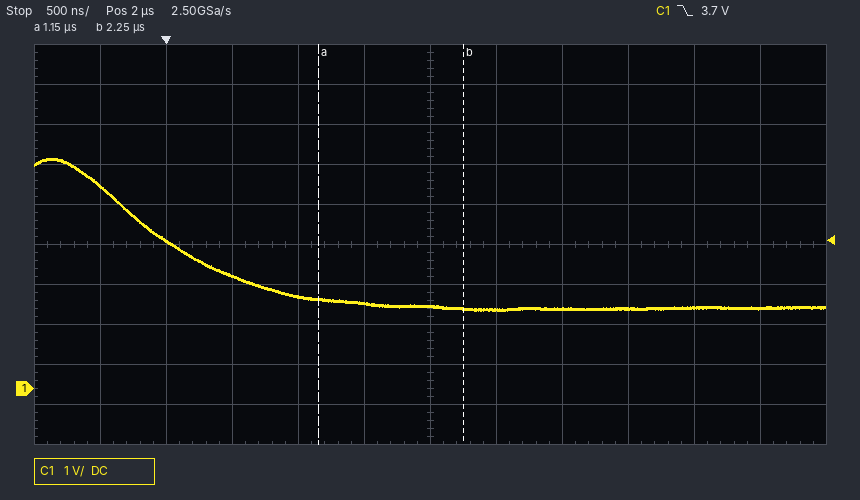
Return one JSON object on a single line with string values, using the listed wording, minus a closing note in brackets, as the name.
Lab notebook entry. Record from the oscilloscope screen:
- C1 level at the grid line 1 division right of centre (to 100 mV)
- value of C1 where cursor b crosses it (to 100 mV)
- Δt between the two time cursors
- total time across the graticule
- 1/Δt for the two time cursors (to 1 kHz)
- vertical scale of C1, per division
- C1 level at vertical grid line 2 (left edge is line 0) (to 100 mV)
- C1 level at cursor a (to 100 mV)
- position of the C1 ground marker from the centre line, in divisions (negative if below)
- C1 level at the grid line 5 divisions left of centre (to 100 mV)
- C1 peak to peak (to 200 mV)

{"C1 level at the grid line 1 division right of centre": "2.0 V", "value of C1 where cursor b crosses it": "2.0 V", "Δt between the two time cursors": "1.10 µs", "total time across the graticule": "6 µs", "1/Δt for the two time cursors": "909 kHz", "vertical scale of C1, per division": "1 V", "C1 level at vertical grid line 2 (left edge is line 0)": "3.7 V", "C1 level at cursor a": "2.2 V", "position of the C1 ground marker from the centre line, in divisions": "-3.6 div", "C1 level at the grid line 5 divisions left of centre": "5.1 V", "C1 peak to peak": "3.8 V"}
